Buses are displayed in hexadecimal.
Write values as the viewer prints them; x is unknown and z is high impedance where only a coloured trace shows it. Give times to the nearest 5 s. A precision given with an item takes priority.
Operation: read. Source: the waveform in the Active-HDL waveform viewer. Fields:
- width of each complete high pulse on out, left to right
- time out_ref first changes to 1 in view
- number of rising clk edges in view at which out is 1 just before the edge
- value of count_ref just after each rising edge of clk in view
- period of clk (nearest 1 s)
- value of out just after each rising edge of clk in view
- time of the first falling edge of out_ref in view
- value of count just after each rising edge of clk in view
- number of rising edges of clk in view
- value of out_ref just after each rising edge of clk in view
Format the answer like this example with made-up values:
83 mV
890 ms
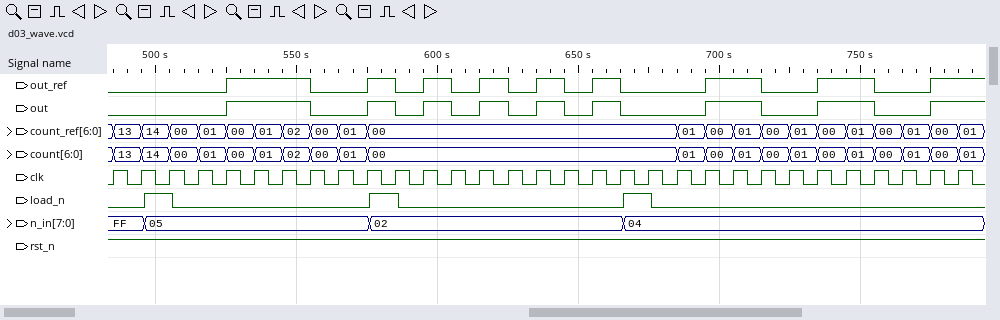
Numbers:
30 s, 10 s, 10 s, 10 s, 10 s, 10 s, 20 s, 20 s
525 s
13
13, 14, 00, 01, 00, 01, 02, 00, 01, 00, 00, 00, 00, 00, 00, 00, 00, 00, 00, 00, 01, 00, 01, 00, 01, 00, 01, 00, 01, 00, 01
10 s
0 0 0 0 1 1 1 0 0 1 0 1 0 1 0 1 0 1 0 0 0 1 1 0 0 1 1 0 0 1 1
555 s
13, 14, 00, 01, 00, 01, 02, 00, 01, 00, 00, 00, 00, 00, 00, 00, 00, 00, 00, 00, 01, 00, 01, 00, 01, 00, 01, 00, 01, 00, 01
31
0 0 0 0 1 1 1 0 0 1 0 1 0 1 0 1 0 1 0 0 0 1 1 0 0 1 1 0 0 1 1
